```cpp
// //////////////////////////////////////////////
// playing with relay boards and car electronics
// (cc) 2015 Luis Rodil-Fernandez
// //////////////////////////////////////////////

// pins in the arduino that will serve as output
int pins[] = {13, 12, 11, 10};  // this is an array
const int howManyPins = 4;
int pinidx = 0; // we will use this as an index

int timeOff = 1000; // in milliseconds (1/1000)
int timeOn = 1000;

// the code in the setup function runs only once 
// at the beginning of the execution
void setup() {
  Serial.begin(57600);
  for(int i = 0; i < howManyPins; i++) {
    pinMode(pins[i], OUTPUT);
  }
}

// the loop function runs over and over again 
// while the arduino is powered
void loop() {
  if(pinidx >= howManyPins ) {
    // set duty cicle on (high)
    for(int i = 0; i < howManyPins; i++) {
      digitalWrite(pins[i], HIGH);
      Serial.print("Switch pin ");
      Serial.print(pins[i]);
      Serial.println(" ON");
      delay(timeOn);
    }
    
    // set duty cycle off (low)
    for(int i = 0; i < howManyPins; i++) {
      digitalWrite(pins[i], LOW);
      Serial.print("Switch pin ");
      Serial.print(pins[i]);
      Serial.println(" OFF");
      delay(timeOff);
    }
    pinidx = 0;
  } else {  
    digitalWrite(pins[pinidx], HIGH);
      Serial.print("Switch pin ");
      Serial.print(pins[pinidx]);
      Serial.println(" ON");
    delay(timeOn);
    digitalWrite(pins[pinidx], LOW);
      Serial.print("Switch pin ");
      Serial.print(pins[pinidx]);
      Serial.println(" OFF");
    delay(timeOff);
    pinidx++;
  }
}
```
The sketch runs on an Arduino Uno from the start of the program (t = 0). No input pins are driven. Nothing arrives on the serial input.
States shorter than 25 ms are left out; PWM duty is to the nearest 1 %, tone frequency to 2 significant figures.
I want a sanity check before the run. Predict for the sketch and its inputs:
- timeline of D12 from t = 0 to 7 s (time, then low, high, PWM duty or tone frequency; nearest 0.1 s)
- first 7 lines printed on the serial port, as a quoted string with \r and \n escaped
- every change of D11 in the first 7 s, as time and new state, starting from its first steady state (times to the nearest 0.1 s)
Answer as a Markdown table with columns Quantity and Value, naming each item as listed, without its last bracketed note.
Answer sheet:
| Quantity | Value |
|---|---|
| timeline of D12 from t = 0 to 7 s | 0 s low; 2 s high; 3 s low |
| first 7 lines printed on the serial port, as a quoted string with \r and \n escaped | "Switch pin 13 ON\r\nSwitch pin 13 OFF\r\nSwitch pin 12 ON\r\nSwitch pin 12 OFF\r\nSwitch pin 11 ON\r\nSwitch pin 11 OFF\r\nSwitch pin 10 ON\r\n" |
| every change of D11 in the first 7 s, as time and new state, starting from its first steady state | 0 s low; 4 s high; 5 s low |
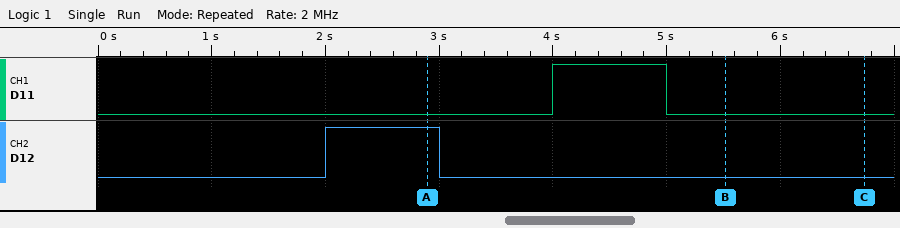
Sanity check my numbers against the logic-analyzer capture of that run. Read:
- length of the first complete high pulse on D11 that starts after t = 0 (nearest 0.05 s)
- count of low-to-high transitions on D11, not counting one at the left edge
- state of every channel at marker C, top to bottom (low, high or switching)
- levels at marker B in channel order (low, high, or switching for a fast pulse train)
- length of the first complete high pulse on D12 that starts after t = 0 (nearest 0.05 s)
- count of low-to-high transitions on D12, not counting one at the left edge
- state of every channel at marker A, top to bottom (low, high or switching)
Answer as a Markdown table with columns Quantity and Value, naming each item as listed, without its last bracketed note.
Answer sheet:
| Quantity | Value |
|---|---|
| length of the first complete high pulse on D11 that starts after t = 0 | 1.00 s |
| count of low-to-high transitions on D11, not counting one at the left edge | 1 |
| state of every channel at marker C, top to bottom | D11 low, D12 low |
| levels at marker B in channel order | D11 low, D12 low |
| length of the first complete high pulse on D12 that starts after t = 0 | 1.00 s |
| count of low-to-high transitions on D12, not counting one at the left edge | 1 |
| state of every channel at marker A, top to bottom | D11 low, D12 high |
